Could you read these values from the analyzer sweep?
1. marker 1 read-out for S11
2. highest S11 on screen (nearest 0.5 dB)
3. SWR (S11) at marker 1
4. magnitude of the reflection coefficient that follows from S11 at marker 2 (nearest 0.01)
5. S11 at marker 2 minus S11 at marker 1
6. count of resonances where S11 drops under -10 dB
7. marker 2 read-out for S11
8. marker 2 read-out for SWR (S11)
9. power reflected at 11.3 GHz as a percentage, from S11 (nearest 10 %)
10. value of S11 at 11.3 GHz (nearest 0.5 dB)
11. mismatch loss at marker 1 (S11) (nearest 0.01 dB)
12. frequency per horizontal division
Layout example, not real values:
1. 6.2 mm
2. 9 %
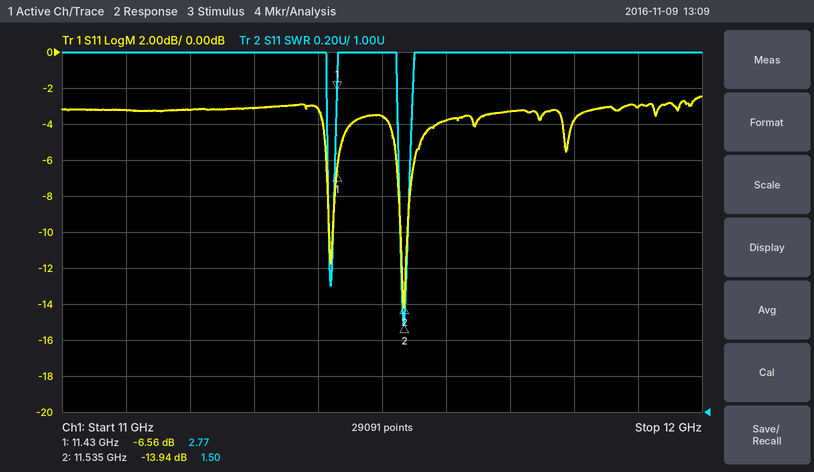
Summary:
1. -6.56 dB
2. -2.5 dB
3. 2.77
4. 0.20
5. -7.38 dB
6. 2
7. -13.94 dB
8. 1.50
9. 50 %
10. -3.0 dB
11. 1.08 dB
12. 100 MHz
